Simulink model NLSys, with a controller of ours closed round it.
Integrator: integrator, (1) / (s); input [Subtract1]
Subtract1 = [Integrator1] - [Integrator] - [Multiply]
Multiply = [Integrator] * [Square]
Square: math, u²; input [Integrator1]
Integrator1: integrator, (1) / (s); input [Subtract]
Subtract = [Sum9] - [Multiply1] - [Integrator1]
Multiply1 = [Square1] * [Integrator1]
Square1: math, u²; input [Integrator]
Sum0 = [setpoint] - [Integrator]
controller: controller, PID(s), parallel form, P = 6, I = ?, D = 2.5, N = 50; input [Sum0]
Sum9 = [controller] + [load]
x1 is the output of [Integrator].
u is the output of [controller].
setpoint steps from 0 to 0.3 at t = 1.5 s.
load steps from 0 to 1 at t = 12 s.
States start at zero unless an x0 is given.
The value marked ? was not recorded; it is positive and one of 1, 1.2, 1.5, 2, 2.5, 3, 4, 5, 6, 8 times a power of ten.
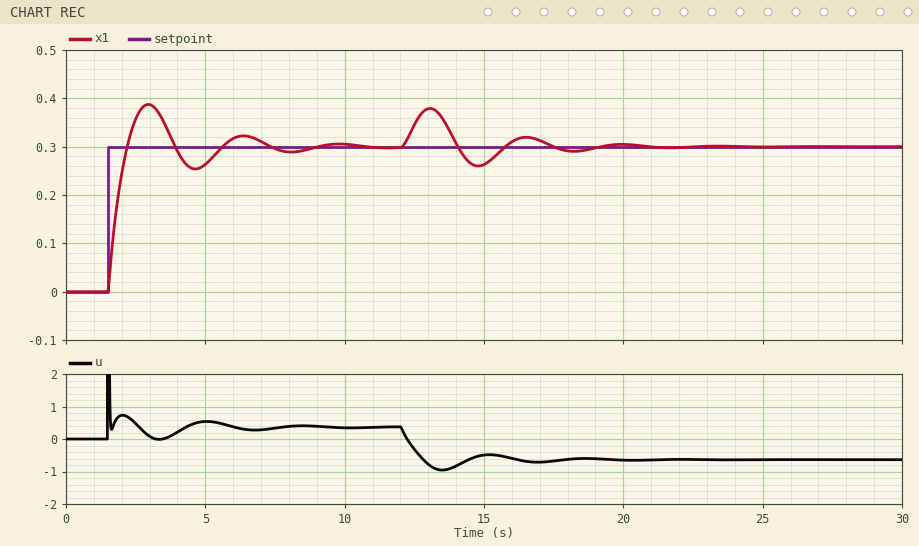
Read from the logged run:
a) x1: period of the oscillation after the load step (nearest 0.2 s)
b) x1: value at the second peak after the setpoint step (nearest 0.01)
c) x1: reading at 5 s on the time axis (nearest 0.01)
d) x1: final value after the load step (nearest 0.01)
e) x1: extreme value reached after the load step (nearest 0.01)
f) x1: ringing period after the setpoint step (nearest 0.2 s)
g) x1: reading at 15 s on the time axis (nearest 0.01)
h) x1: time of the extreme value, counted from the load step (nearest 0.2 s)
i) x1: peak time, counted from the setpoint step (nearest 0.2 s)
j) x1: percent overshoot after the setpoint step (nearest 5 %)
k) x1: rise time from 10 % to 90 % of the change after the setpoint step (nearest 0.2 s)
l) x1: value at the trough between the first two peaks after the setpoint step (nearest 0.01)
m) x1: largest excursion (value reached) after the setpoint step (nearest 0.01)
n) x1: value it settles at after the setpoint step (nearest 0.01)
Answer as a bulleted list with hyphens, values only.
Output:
- 3.4 s
- 0.32
- 0.26
- 0.30
- 0.38
- 3.4 s
- 0.26
- 1.0 s
- 1.4 s
- 30 %
- 0.6 s
- 0.25
- 0.39
- 0.30
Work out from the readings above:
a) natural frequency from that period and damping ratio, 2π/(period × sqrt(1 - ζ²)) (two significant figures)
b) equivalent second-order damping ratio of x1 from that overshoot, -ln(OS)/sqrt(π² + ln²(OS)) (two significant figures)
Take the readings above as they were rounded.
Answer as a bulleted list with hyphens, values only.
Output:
- 2.0 rad/s
- 0.36
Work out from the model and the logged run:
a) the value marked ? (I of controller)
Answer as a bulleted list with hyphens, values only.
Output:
- 15
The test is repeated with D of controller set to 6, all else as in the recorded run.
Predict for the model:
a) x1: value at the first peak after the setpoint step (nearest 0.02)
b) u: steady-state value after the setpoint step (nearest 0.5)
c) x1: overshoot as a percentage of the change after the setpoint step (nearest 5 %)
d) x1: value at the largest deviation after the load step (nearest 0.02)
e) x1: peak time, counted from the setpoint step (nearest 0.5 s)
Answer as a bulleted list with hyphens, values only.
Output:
- 0.34
- 0.5
- 15 %
- 0.36
- 2.0 s
